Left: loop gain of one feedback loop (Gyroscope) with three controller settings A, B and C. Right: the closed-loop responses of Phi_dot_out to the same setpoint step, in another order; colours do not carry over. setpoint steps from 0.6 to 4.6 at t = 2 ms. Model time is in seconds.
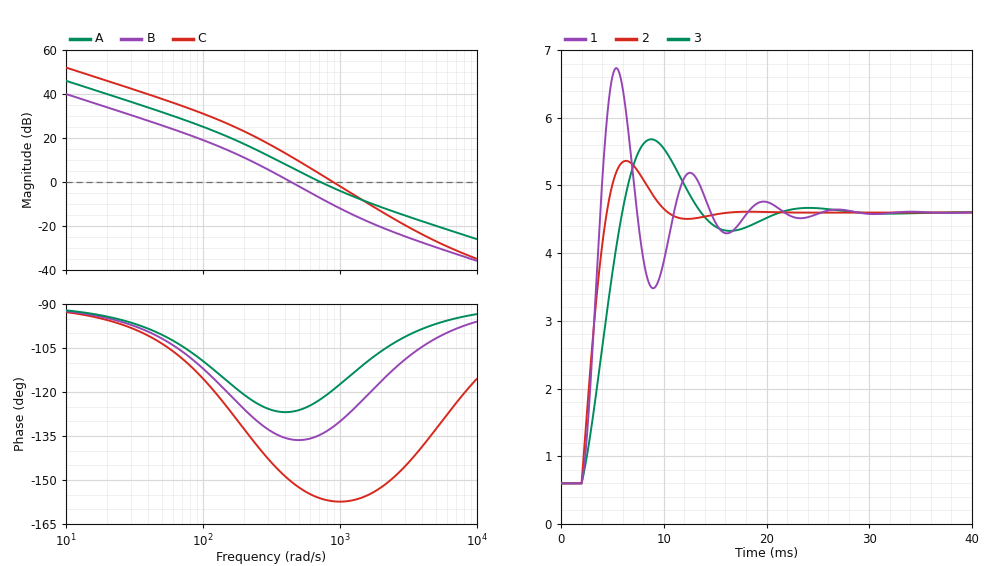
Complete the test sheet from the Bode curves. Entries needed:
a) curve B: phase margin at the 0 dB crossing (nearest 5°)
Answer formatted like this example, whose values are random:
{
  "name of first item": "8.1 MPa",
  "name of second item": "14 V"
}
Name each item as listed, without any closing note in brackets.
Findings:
{
  "curve B: phase margin at the 0 dB crossing": "45°"
}
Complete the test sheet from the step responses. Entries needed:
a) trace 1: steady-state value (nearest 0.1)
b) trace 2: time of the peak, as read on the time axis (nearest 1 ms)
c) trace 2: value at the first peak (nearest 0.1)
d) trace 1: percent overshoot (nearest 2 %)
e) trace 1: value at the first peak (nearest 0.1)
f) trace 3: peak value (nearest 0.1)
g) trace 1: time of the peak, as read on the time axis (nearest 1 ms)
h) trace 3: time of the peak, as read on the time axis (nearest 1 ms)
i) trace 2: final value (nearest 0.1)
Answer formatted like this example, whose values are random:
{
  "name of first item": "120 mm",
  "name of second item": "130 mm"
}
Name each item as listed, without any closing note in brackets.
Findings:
{
  "trace 1: steady-state value": "4.6",
  "trace 2: time of the peak, as read on the time axis": "6 ms",
  "trace 2: value at the first peak": "5.4",
  "trace 1: percent overshoot": "54 %",
  "trace 1: value at the first peak": "6.7",
  "trace 3: peak value": "5.7",
  "trace 1: time of the peak, as read on the time axis": "5 ms",
  "trace 3: time of the peak, as read on the time axis": "9 ms",
  "trace 2: final value": "4.6"
}
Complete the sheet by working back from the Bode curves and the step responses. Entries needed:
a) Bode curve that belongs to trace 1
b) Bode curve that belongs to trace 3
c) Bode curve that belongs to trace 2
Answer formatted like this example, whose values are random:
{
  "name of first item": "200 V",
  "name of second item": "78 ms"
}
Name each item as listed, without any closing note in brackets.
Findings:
{
  "Bode curve that belongs to trace 1": "C",
  "Bode curve that belongs to trace 3": "B",
  "Bode curve that belongs to trace 2": "A"
}
